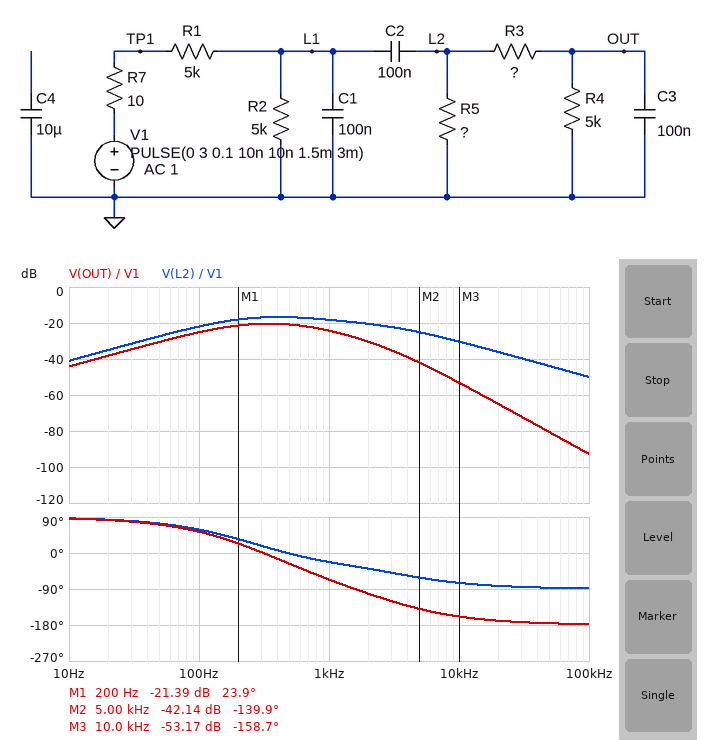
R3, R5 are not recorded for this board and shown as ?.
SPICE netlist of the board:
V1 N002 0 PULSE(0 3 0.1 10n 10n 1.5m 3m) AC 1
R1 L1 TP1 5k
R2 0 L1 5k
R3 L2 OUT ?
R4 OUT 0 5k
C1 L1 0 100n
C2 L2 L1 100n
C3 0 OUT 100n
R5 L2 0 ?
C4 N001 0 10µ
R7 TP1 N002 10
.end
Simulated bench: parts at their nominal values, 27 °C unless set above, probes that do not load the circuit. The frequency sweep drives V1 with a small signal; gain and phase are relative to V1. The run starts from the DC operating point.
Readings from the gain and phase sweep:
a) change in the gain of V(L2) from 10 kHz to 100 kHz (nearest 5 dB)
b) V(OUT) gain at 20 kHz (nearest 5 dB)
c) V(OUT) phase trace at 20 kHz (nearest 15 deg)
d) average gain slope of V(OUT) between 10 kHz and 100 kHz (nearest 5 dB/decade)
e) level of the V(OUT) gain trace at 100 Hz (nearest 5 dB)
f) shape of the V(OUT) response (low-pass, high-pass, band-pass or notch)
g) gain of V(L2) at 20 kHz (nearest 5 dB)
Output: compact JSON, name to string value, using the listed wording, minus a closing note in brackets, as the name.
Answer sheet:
{"change in the gain of V(L2) from 10 kHz to 100 kHz": "-20 dB", "V(OUT) gain at 20 kHz": "-65 dB", "V(OUT) phase trace at 20 kHz": "-165 deg", "average gain slope of V(OUT) between 10 kHz and 100 kHz": "-40 dB/decade", "level of the V(OUT) gain trace at 100 Hz": "-25 dB", "shape of the V(OUT) response": "band-pass", "gain of V(L2) at 20 kHz": "-35 dB"}
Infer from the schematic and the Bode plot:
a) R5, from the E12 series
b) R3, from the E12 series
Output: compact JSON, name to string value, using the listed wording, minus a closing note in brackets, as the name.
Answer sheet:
{"R5, from the E12 series": "4.7 kΩ", "R3, from the E12 series": "2.2 kΩ"}
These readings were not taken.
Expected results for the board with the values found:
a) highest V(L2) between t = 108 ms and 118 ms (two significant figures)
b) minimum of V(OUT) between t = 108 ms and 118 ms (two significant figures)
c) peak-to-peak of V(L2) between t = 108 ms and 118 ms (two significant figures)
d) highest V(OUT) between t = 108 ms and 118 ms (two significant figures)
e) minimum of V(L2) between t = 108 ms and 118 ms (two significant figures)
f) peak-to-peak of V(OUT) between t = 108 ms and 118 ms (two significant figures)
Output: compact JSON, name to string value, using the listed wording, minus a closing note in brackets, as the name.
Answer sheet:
{"highest V(L2) between t = 108 ms and 118 ms": "290 mV", "minimum of V(OUT) between t = 108 ms and 118 ms": "-180 mV", "peak-to-peak of V(L2) between t = 108 ms and 118 ms": "580 mV", "highest V(OUT) between t = 108 ms and 118 ms": "180 mV", "minimum of V(L2) between t = 108 ms and 118 ms": "-290 mV", "peak-to-peak of V(OUT) between t = 108 ms and 118 ms": "360 mV"}
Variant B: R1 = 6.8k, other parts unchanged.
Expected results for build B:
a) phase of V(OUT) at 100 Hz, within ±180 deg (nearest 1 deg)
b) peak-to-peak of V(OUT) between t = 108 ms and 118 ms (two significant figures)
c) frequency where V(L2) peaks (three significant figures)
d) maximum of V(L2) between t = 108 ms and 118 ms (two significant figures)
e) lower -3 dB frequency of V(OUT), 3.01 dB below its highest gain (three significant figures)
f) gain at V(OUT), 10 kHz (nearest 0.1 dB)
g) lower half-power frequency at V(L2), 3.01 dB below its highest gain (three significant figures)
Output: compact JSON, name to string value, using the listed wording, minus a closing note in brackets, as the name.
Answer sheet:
{"phase of V(OUT) at 100 Hz, within ±180 deg": "51 deg", "peak-to-peak of V(OUT) between t = 108 ms and 118 ms": "280 mV", "frequency where V(L2) peaks": "374 Hz", "maximum of V(L2) between t = 108 ms and 118 ms": "220 mV", "lower -3 dB frequency of V(OUT), 3.01 dB below its highest gain": "123 Hz", "gain at V(OUT), 10 kHz": "-55.8 dB", "lower half-power frequency at V(L2), 3.01 dB below its highest gain": "132 Hz"}
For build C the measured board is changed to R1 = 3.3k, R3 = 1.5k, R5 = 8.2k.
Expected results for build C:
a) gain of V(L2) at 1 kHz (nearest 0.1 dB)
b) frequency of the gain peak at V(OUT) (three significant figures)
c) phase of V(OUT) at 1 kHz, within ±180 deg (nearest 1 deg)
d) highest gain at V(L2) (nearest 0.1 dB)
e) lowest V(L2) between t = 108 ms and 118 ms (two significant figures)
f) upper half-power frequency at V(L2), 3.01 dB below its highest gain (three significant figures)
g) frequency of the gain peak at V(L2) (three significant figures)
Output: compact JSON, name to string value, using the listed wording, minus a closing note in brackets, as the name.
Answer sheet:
{"gain of V(L2) at 1 kHz": "-15.4 dB", "frequency of the gain peak at V(OUT)": "350 Hz", "phase of V(OUT) at 1 kHz, within ±180 deg": "-61 deg", "highest gain at V(L2)": "-13.4 dB", "lowest V(L2) between t = 108 ms and 118 ms": "-410 mV", "upper half-power frequency at V(L2), 3.01 dB below its highest gain": "1.34 kHz", "frequency of the gain peak at V(L2)": "385 Hz"}
